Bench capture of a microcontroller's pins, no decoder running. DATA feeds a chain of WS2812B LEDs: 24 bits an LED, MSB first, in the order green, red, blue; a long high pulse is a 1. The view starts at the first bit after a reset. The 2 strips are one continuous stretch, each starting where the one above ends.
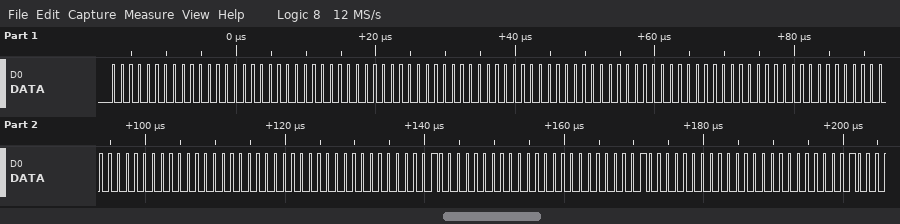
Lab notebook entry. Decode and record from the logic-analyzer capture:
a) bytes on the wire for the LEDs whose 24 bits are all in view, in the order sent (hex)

00 00 00 00 00 00 00 00 00 00 00 00 00 00 00 01 00 00 01 00 00
